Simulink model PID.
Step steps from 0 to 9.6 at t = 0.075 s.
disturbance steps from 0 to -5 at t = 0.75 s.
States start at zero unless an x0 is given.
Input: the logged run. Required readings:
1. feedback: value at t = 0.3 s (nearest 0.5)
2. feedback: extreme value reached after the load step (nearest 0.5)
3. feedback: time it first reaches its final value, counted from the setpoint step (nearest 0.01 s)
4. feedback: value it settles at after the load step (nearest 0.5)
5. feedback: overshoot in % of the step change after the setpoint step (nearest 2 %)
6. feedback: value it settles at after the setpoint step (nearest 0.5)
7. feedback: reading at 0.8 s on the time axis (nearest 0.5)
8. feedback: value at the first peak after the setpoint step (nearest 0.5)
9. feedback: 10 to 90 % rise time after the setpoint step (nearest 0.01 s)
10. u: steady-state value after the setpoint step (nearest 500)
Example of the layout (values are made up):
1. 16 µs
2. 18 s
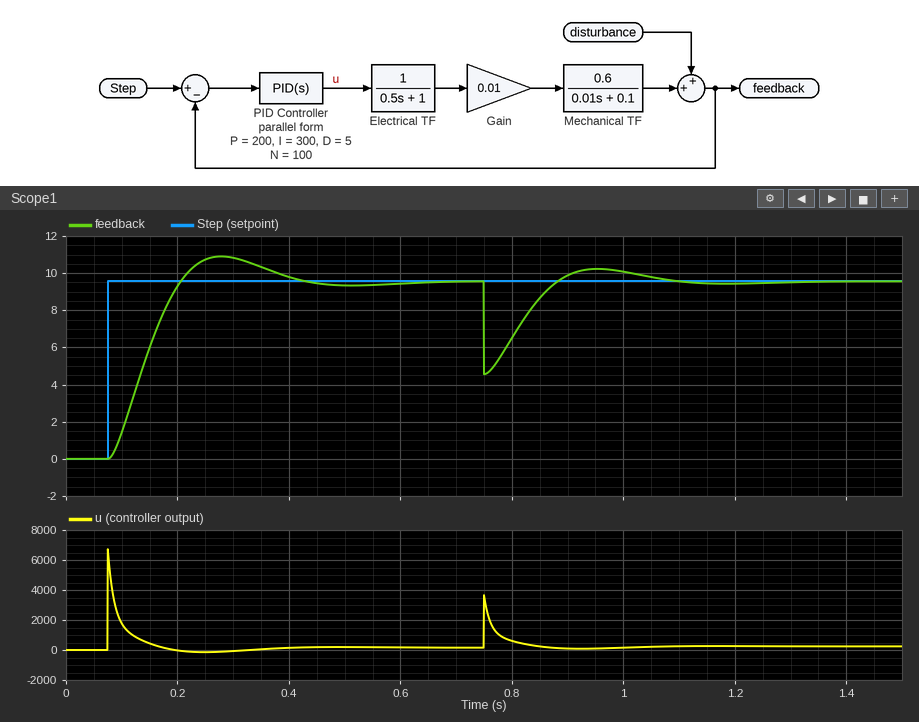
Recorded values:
1. 11.0
2. 4.5
3. 0.13 s
4. 9.5
5. 14 %
6. 9.5
7. 6.5
8. 11.0
9. 0.09 s
10. 0
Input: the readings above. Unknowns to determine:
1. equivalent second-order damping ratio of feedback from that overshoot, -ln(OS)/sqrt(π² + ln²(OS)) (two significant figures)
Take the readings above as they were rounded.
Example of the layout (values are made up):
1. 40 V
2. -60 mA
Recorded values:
1. 0.53
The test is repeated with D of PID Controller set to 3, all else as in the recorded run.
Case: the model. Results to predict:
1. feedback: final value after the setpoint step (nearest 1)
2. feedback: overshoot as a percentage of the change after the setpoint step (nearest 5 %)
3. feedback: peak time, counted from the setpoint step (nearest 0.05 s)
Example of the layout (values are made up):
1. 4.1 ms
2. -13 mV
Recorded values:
1. 10
2. 20 %
3. 0.20 s
